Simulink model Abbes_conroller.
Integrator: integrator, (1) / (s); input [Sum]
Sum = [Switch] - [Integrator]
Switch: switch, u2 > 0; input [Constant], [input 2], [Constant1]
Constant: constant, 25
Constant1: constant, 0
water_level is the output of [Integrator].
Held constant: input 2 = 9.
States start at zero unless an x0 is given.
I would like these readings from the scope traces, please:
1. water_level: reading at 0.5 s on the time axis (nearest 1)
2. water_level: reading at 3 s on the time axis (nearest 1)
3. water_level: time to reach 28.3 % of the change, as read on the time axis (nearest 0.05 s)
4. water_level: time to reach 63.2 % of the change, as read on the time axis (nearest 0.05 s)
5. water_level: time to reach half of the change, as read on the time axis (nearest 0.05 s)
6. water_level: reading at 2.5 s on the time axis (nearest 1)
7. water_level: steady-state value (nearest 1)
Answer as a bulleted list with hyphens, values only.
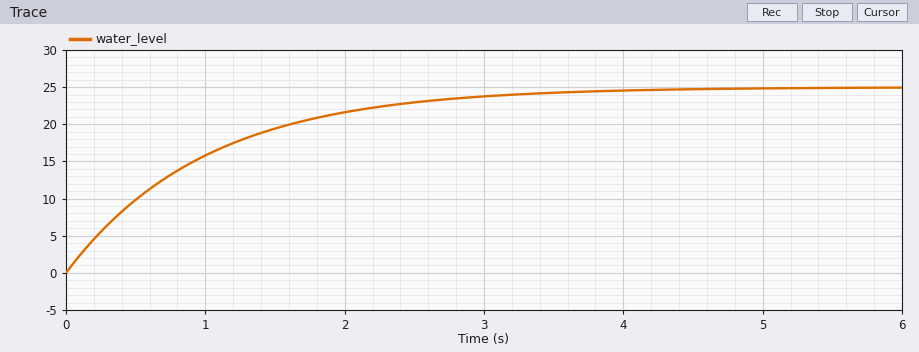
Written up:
- 10
- 24
- 0.35 s
- 1.00 s
- 0.70 s
- 23
- 25
